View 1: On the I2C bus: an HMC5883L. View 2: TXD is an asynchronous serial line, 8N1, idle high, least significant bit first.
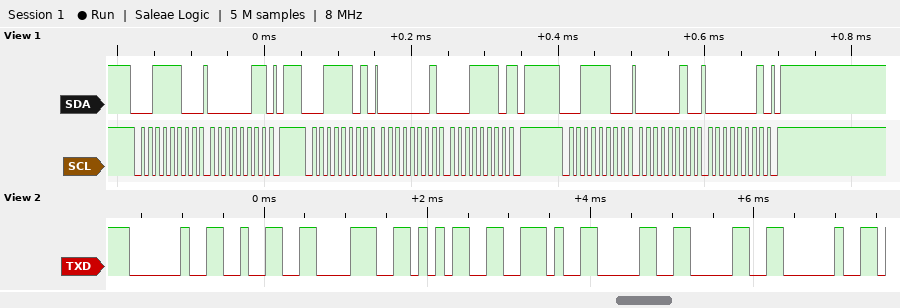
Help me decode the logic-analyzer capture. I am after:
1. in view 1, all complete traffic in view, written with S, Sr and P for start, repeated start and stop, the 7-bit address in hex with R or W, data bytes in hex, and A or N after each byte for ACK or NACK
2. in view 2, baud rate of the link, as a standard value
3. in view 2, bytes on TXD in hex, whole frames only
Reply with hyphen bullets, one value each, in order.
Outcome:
- S 1EW A 03 A P S 1ER A 01 A 1E N P S 1EW A 02 A 01 A P
- 9600 baud
- 0x20 0x32 0x38 0x35 0x2E 0x30 0x30 0x20
